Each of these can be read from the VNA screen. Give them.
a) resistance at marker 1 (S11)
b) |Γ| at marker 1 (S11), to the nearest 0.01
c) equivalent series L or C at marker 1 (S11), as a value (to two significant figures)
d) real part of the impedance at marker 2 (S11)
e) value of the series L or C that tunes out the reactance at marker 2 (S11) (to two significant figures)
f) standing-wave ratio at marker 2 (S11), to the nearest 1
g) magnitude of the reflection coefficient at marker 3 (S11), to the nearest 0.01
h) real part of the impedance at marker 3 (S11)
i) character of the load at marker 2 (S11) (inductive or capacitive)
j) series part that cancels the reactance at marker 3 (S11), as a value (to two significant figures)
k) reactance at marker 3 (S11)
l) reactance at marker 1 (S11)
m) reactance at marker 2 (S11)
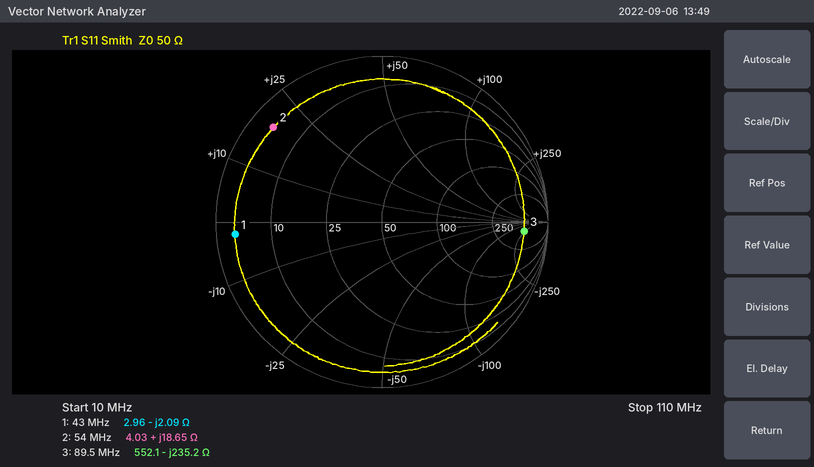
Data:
2.96 Ω
0.89
1.8 nF
4.03 Ω
160 pF
14
0.86
552.1 Ω
inductive
420 nH
-235.2 Ω
-2.09 Ω
+18.65 Ω
